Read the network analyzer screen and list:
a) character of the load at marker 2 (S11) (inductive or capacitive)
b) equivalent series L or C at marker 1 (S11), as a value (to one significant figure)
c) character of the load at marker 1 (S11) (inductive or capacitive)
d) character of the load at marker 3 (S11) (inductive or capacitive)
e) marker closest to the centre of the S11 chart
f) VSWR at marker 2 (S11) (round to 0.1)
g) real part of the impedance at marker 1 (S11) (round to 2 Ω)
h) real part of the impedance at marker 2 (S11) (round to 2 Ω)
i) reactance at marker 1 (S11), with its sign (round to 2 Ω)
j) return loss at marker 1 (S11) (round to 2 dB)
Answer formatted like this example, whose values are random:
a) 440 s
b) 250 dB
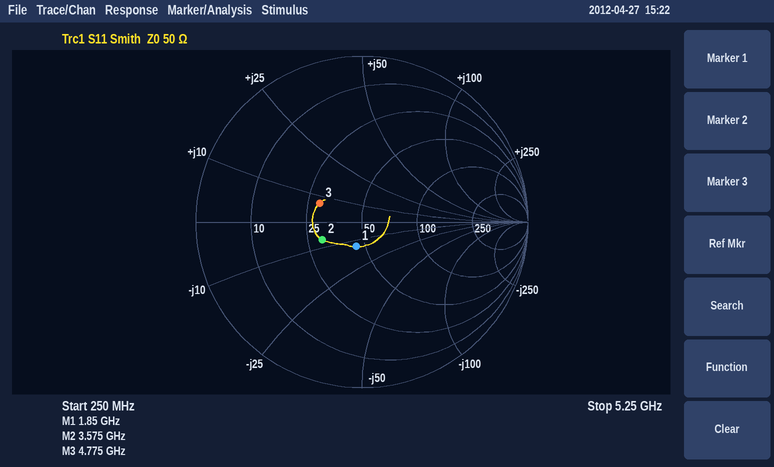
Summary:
a) capacitive
b) 6 pF
c) capacitive
d) inductive
e) marker 1
f) 1.7
g) 44 Ω
h) 30 Ω
i) -14 Ω
j) 16 dB
